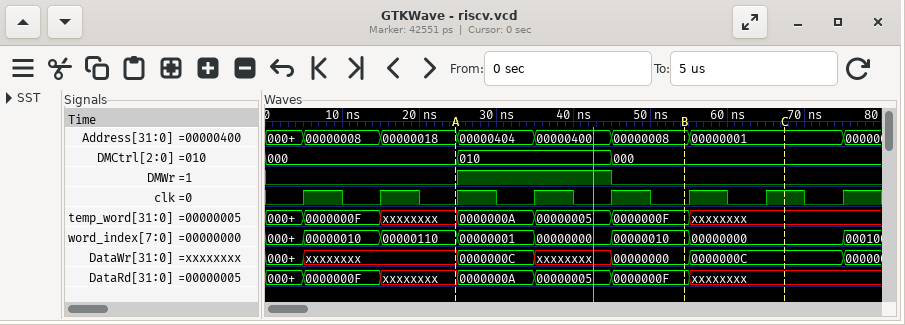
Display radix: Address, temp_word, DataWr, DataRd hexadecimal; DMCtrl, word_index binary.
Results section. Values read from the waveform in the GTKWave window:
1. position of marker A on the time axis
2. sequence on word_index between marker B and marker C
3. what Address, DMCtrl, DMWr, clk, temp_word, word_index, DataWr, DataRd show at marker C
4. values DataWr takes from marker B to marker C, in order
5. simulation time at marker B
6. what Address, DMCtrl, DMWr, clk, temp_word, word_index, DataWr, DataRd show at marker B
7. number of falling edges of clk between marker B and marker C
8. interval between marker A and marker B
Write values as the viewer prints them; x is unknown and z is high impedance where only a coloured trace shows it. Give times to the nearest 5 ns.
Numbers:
25 ns
00000010, 00000000
Address=00000001, DMCtrl=000, DMWr=0, clk=1, temp_word=xxxxxxxx, word_index=00000000, DataWr=0000000C, DataRd=xxxxxxxx
00000000, 0000000C
55 ns
Address=00000008, DMCtrl=000, DMWr=0, clk=0, temp_word=0000000F, word_index=00000010, DataWr=00000000, DataRd=0000000F
1
30 ns
